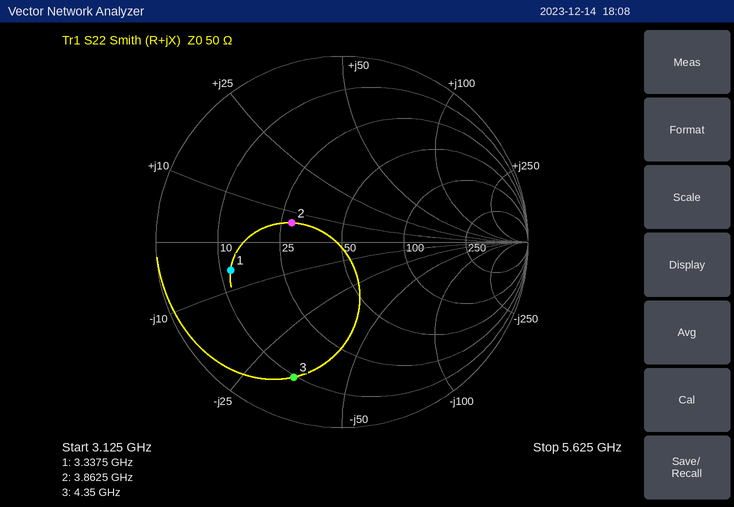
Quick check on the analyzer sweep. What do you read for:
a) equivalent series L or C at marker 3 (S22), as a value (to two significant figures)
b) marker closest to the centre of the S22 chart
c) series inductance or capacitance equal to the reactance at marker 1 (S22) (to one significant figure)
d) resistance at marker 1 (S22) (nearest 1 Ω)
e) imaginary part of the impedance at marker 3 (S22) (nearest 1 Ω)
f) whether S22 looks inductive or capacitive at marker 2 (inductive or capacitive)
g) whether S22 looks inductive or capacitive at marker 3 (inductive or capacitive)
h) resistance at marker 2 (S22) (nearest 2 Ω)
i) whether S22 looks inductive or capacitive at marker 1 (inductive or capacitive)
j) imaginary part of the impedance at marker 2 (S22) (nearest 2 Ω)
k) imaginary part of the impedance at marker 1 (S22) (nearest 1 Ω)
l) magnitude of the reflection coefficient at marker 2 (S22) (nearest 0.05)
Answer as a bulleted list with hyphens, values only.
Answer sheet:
- 1.1 pF
- marker 2
- 8 pF
- 12 Ω
- -34 Ω
- inductive
- capacitive
- 28 Ω
- capacitive
- +6 Ω
- -6 Ω
- 0.30
